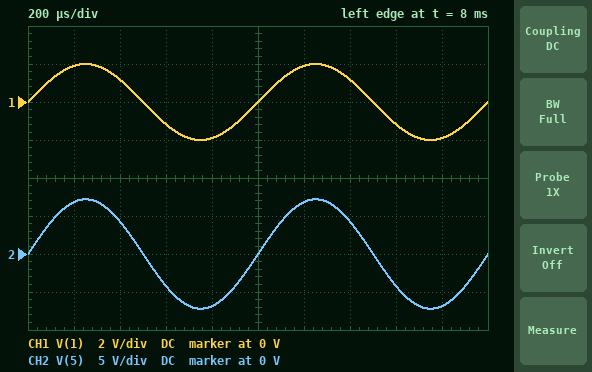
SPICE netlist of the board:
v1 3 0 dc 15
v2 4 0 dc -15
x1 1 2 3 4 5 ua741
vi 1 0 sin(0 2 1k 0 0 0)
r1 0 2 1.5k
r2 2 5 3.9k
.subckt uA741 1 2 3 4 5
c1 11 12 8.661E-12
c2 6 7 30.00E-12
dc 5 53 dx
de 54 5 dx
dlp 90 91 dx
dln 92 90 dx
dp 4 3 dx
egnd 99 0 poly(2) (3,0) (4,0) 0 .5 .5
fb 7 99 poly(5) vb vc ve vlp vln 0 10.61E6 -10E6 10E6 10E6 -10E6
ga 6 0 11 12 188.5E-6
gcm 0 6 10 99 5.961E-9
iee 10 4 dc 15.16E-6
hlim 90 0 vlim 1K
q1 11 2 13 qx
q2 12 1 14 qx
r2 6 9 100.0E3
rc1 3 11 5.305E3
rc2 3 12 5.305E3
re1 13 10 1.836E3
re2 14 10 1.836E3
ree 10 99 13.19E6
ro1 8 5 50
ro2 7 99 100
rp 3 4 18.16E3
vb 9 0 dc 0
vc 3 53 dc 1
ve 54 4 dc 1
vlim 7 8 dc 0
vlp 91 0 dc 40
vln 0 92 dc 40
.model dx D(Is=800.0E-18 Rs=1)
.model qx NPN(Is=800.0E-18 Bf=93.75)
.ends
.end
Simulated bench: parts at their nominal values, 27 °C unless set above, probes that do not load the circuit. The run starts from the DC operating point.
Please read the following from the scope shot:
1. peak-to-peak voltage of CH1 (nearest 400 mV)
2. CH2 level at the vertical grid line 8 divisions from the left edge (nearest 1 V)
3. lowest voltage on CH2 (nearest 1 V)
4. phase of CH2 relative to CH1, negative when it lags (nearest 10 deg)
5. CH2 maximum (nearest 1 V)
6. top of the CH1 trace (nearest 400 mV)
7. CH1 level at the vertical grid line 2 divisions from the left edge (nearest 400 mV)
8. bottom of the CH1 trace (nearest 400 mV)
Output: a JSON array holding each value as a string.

["4.0 V", "-4 V", "-7 V", "0 deg", "7 V", "2.0 V", "1.2 V", "-2.0 V"]
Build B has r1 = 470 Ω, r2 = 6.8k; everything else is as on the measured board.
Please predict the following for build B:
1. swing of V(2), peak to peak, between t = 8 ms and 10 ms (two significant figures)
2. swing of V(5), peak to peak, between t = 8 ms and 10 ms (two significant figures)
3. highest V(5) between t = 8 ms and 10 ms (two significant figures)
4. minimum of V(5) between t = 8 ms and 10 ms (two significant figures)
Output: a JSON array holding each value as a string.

["1.9 V", "29 V", "15 V", "-15 V"]
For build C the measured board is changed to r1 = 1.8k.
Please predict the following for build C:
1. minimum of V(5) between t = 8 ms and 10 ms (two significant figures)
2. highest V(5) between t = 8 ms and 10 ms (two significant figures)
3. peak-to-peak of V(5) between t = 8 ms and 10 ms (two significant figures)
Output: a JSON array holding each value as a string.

["-6.3 V", "6.3 V", "13 V"]
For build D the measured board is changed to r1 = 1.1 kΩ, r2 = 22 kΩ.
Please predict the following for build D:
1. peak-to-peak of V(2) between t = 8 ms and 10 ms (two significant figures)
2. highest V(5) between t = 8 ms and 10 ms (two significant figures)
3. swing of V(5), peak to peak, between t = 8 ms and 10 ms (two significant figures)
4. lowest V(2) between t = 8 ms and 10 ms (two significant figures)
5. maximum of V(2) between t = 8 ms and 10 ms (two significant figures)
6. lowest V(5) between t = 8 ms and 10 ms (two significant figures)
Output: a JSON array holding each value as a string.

["1.4 V", "15 V", "29 V", "-700 mV", "700 mV", "-15 V"]
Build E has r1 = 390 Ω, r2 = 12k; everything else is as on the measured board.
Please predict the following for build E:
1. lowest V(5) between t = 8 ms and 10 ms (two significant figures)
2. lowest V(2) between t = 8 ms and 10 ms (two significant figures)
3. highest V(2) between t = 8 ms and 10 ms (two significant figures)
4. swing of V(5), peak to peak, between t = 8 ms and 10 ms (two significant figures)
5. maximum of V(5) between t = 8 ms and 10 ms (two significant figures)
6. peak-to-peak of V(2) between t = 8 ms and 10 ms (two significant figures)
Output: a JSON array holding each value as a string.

["-15 V", "-460 mV", "460 mV", "29 V", "15 V", "920 mV"]
